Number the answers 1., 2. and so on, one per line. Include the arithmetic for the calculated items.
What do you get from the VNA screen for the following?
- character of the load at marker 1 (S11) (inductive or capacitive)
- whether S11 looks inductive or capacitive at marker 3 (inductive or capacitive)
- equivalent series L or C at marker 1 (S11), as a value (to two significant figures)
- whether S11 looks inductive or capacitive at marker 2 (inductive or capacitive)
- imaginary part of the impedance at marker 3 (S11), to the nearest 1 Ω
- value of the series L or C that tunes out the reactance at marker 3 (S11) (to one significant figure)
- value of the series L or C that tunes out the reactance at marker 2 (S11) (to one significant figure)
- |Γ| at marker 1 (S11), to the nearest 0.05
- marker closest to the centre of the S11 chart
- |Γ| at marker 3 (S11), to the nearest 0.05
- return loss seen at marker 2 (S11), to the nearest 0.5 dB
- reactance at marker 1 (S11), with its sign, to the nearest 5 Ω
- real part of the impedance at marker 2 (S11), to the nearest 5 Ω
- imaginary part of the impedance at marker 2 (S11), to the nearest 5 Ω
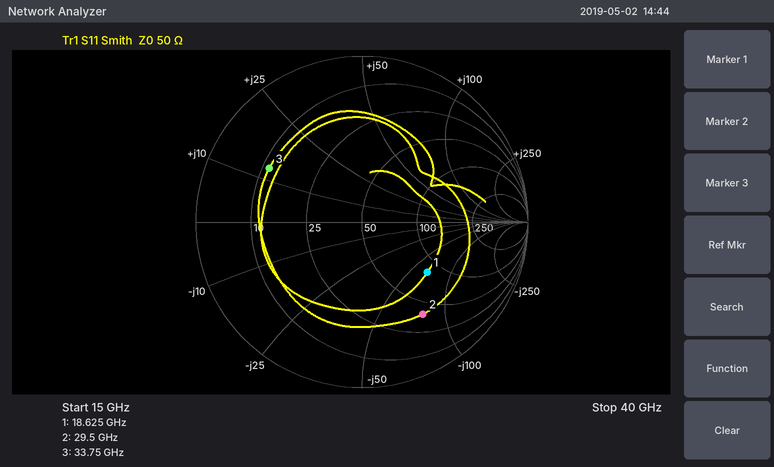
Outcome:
1. capacitive
2. inductive
3. C = 1/(2π × 18.625 GHz × 65 Ω) ≈ 131 fF, so 130 fF to two significant figures
4. capacitive
5. +13 Ω
6. C = 1/(2π × 33.75 GHz × 13 Ω) ≈ 363 fF, so 400 fF to one significant figure
7. L = 80 Ω/(2π × 29.5 GHz) ≈ 432 pH, so 400 pH to one significant figure
8. 0.50
9. marker 1
10. 0.65
11. 3.5 dB
12. -65 Ω
13. 40 Ω
14. -80 Ω
